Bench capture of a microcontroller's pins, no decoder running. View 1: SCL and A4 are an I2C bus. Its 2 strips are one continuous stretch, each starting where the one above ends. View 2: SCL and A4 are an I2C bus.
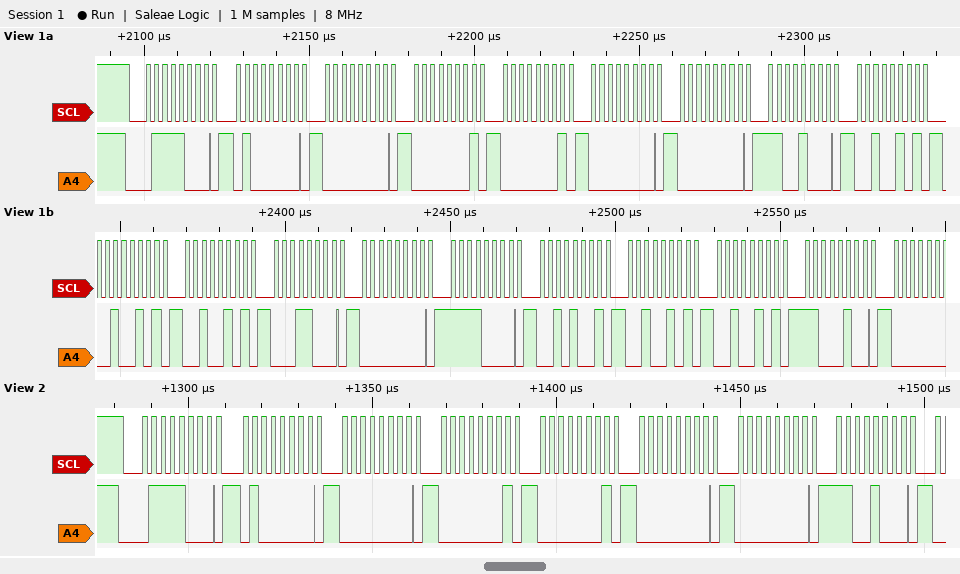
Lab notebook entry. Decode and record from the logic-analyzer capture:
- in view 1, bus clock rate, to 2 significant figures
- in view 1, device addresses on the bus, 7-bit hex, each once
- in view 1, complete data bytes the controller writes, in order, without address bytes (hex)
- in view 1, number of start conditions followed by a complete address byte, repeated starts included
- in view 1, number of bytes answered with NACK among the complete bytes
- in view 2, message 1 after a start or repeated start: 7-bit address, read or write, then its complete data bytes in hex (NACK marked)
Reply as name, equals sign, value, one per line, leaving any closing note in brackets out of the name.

in view 1, bus clock rate, to 2 significant figures = 400 kHz
in view 1, device addresses on the bus, 7-bit hex, each once = 0x3C
in view 1, complete data bytes the controller writes, in order, without address bytes = 40 00 01 01 00 00 C8 25 25 25 18 00 F0 29 25 25 C4
in view 1, number of start conditions followed by a complete address byte, repeated starts included = 1
in view 1, number of bytes answered with NACK among the complete bytes = 0
in view 2, message 1 after a start or repeated start: 7-bit address, read or write, then its complete data bytes in hex = 0x3C write: 40 00 01 01 00 00 C8
